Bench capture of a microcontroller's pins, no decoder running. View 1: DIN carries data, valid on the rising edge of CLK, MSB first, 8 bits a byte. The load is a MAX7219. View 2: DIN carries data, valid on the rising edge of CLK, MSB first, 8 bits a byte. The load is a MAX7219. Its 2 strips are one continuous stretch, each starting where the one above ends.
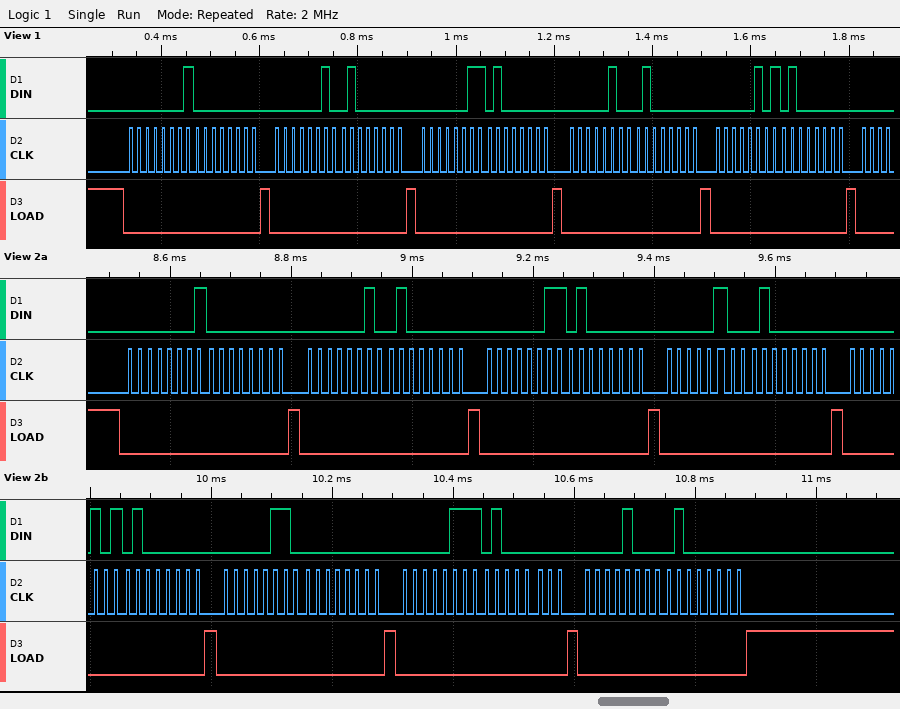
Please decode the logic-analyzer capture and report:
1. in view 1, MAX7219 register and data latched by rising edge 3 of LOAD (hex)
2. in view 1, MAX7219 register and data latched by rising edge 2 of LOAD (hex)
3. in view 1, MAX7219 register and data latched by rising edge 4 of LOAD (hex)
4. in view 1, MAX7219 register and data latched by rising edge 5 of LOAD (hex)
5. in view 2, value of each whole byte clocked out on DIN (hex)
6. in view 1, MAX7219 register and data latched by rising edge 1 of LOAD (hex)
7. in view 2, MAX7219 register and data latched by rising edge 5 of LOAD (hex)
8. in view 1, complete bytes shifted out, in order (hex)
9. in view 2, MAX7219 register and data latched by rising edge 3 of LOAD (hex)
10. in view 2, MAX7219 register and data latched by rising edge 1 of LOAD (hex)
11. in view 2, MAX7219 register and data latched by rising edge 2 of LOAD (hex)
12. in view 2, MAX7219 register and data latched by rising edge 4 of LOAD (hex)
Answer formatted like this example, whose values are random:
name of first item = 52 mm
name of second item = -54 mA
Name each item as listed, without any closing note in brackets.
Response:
in view 1, MAX7219 register and data latched by rising edge 3 of LOAD = register 0x3, data 0x40
in view 1, MAX7219 register and data latched by rising edge 2 of LOAD = register 0x2, data 0x40
in view 1, MAX7219 register and data latched by rising edge 4 of LOAD = register 0x4, data 0x40
in view 1, MAX7219 register and data latched by rising edge 5 of LOAD = register 0x5, data 0x40
in view 2, value of each whole byte clocked out on DIN = 01 00 02 40 03 40 04 40 05 40 06 00 07 40 08 40
in view 1, MAX7219 register and data latched by rising edge 1 of LOAD = register 0x1, data 0x00
in view 2, MAX7219 register and data latched by rising edge 5 of LOAD = register 0x5, data 0x40
in view 1, complete bytes shifted out, in order = 01 00 02 40 03 40 04 40 05 40
in view 2, MAX7219 register and data latched by rising edge 3 of LOAD = register 0x3, data 0x40
in view 2, MAX7219 register and data latched by rising edge 1 of LOAD = register 0x1, data 0x00
in view 2, MAX7219 register and data latched by rising edge 2 of LOAD = register 0x2, data 0x40
in view 2, MAX7219 register and data latched by rising edge 4 of LOAD = register 0x4, data 0x40
